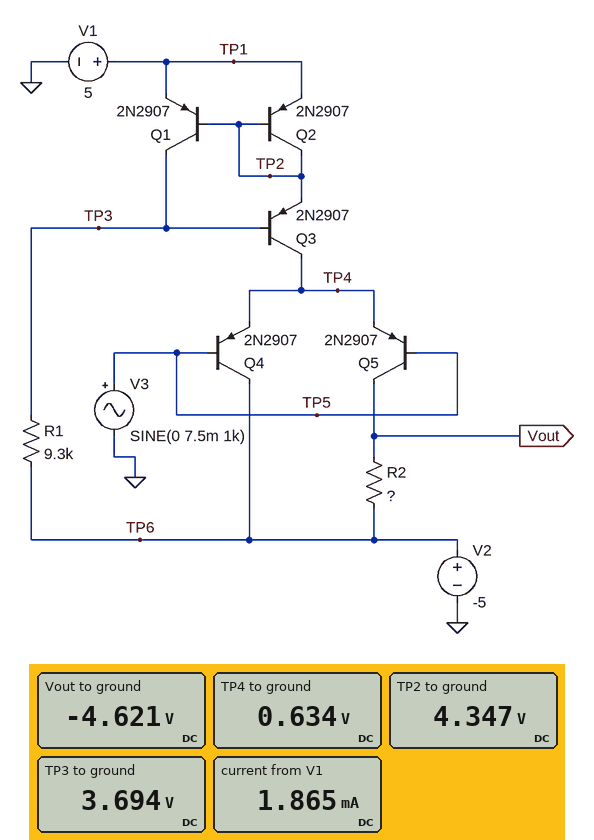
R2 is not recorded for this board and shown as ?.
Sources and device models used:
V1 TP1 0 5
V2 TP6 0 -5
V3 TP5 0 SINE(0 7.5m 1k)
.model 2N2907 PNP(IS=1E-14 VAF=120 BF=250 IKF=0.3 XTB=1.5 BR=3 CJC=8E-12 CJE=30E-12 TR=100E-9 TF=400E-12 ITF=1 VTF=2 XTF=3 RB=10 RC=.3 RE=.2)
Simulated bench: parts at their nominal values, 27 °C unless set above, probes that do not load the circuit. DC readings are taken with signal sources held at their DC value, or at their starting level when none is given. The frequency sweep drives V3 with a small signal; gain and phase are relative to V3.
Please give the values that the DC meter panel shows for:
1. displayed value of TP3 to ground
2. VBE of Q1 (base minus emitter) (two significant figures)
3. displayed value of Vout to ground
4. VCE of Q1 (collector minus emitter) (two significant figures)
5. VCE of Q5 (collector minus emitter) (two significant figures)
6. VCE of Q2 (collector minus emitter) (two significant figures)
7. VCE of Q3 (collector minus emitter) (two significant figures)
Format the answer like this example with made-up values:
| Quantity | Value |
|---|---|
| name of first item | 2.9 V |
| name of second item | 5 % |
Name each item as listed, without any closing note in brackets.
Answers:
| Quantity | Value |
|---|---|
| displayed value of TP3 to ground | 3.694 V |
| VBE of Q1 (base minus emitter) | -650 mV |
| displayed value of Vout to ground | -4.621 V |
| VCE of Q1 (collector minus emitter) | -1.3 V |
| VCE of Q5 (collector minus emitter) | -5.3 V |
| VCE of Q2 (collector minus emitter) | -650 mV |
| VCE of Q3 (collector minus emitter) | -3.7 V |
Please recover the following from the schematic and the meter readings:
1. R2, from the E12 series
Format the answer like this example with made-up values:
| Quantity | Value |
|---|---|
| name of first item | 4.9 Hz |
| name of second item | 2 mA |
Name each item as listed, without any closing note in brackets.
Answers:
| Quantity | Value |
|---|---|
| R2, from the E12 series | 820 Ω |
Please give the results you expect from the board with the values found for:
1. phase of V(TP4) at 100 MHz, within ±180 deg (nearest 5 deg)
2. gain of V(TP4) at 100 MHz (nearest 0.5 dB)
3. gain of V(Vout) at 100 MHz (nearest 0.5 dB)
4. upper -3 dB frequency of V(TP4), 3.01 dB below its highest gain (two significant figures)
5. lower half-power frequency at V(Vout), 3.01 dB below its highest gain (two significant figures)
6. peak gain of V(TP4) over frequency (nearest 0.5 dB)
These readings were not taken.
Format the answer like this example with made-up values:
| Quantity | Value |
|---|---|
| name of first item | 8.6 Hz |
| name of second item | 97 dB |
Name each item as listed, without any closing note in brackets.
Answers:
| Quantity | Value |
|---|---|
| phase of V(TP4) at 100 MHz, within ±180 deg | 0 deg |
| gain of V(TP4) at 100 MHz | -0.5 dB |
| gain of V(Vout) at 100 MHz | -1.0 dB |
| upper -3 dB frequency of V(TP4), 3.01 dB below its highest gain | 3.4 GHz |
| lower half-power frequency at V(Vout), 3.01 dB below its highest gain | 53 MHz |
| peak gain of V(TP4) over frequency | 0 dB |
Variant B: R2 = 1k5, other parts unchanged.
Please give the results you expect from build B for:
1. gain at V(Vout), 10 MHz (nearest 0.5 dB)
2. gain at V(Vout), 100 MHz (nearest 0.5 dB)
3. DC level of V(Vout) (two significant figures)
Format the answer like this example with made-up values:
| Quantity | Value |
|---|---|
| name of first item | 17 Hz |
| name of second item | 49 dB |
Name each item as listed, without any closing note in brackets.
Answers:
| Quantity | Value |
|---|---|
| gain at V(Vout), 10 MHz | -21.0 dB |
| gain at V(Vout), 100 MHz | -0.5 dB |
| DC level of V(Vout) | -4.3 V |
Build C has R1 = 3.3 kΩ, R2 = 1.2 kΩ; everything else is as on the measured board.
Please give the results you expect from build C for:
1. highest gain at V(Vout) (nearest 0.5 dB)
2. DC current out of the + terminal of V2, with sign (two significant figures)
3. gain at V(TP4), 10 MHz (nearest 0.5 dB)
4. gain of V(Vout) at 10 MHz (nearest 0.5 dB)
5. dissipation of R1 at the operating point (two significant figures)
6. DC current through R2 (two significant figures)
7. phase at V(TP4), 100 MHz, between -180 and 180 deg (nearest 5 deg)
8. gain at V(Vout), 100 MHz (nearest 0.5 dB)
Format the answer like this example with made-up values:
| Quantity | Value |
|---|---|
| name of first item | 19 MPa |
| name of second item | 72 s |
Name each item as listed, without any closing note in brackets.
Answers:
| Quantity | Value |
|---|---|
| highest gain at V(Vout) | -0.5 dB |
| DC current out of the + terminal of V2, with sign | -5.2 mA |
| gain at V(TP4), 10 MHz | 0 dB |
| gain of V(Vout) at 10 MHz | -30.5 dB |
| dissipation of R1 at the operating point | 23 mW |
| DC current through R2 | 1.3 mA |
| phase at V(TP4), 100 MHz, between -180 and 180 deg | -5 deg |
| gain at V(Vout), 100 MHz | -2.5 dB |
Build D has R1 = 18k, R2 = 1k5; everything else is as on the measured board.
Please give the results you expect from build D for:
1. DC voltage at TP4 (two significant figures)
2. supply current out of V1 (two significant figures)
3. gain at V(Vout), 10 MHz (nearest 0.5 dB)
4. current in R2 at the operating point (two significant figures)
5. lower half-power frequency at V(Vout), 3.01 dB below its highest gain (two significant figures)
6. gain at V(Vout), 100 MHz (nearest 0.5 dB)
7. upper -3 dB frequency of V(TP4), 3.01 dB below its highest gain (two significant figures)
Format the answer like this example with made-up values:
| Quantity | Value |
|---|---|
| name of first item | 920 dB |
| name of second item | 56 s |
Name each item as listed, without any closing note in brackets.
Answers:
| Quantity | Value |
|---|---|
| DC voltage at TP4 | 620 mV |
| supply current out of V1 | 970 µA |
| gain at V(Vout), 10 MHz | -16.0 dB |
| current in R2 at the operating point | 240 µA |
| lower half-power frequency at V(Vout), 3.01 dB below its highest gain | 29 MHz |
| gain at V(Vout), 100 MHz | -0.5 dB |
| upper -3 dB frequency of V(TP4), 3.01 dB below its highest gain | 3.5 GHz |
